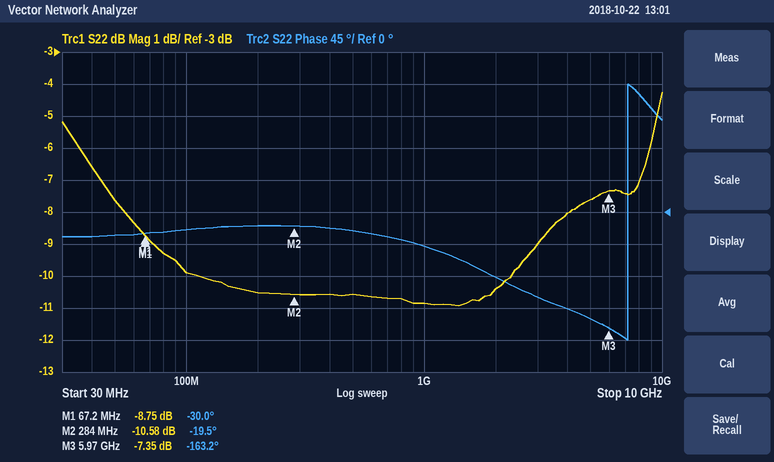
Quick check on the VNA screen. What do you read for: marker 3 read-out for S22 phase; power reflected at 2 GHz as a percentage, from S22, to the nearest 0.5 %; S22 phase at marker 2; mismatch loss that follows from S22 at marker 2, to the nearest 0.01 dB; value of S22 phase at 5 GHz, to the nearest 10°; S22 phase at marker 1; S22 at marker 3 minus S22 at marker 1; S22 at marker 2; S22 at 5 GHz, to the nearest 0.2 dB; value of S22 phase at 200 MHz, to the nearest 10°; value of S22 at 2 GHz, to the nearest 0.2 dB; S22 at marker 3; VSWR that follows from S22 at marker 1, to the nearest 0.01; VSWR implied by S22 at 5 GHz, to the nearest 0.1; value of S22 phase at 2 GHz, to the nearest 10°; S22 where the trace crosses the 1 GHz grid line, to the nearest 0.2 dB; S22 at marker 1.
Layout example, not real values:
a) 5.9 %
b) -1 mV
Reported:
a) -163.2°
b) 9.0 %
c) -19.5°
d) 0.40 dB
e) -150°
f) -30.0°
g) 1.40 dB
h) -10.58 dB
i) -7.6 dB
j) -20°
k) -10.4 dB
l) -7.35 dB
m) 2.15
n) 2.4
o) -90°
p) -10.8 dB
q) -8.75 dB
